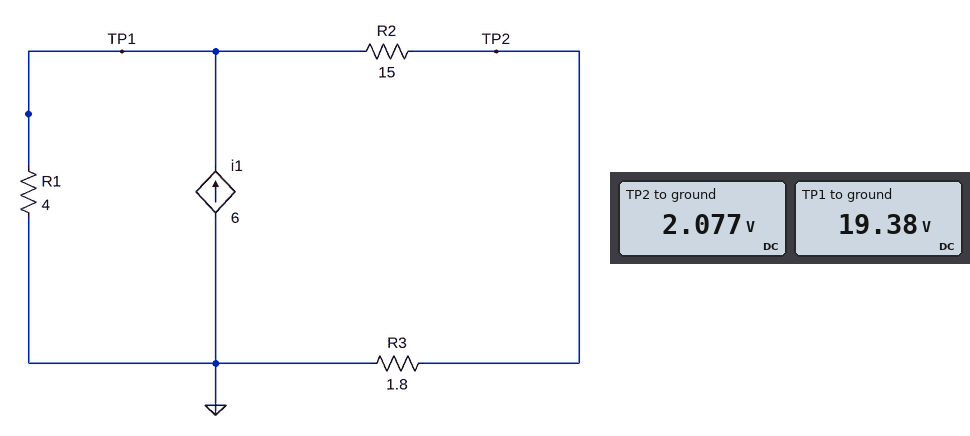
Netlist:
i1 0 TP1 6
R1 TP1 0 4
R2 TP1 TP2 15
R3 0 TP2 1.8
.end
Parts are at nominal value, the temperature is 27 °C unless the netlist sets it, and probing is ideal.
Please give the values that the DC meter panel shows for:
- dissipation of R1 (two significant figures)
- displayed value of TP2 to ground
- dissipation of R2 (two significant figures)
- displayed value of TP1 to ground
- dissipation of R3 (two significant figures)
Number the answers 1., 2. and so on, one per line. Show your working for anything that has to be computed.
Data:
1. (19.38 V)^2 / 4 Ω = 94 W
2. 2.077 V
3. (19.38 V - 2.077 V)^2 / 15 Ω = 20 W
4. 19.38 V
5. (2.077 V)^2 / 1.8 Ω = 2.4 W
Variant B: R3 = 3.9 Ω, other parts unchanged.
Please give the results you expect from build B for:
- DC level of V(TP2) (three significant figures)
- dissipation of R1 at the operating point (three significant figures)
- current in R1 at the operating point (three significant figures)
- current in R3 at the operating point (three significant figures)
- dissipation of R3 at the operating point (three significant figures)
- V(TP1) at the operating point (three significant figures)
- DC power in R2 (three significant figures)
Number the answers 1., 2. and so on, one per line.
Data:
1. 4.09 V
2. 98.1 W
3. 4.95 A
4. 1.05 A
5. 4.28 W
6. 19.8 V
7. 16.5 W
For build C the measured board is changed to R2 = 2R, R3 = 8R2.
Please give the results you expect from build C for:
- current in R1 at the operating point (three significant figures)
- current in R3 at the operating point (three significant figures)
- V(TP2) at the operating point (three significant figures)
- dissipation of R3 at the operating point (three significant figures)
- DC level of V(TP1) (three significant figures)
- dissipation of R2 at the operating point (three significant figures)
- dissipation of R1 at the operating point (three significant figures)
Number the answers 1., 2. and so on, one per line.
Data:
1. 4.31 A
2. 1.69 A
3. 13.9 V
4. 23.4 W
5. 17.2 V
6. 5.71 W
7. 74.3 W
